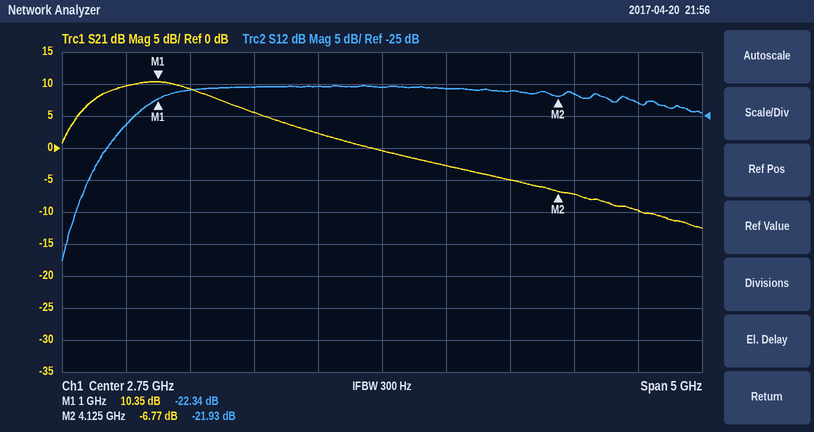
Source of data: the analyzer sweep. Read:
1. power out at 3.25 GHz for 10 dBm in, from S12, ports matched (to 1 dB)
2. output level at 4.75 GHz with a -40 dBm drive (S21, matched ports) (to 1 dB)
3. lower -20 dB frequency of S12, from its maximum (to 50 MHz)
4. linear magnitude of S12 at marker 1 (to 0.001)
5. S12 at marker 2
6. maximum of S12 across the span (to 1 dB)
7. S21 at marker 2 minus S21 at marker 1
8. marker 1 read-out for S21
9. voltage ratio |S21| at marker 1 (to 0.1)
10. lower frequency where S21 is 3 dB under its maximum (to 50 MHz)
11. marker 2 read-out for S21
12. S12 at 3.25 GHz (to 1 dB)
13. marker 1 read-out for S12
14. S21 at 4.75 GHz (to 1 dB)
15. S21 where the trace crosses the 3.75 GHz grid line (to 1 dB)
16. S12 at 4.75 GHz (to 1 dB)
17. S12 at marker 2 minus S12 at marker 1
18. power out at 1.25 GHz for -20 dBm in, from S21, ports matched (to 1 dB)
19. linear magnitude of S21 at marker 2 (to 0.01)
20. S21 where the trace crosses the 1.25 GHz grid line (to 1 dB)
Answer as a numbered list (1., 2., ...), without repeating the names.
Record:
1. -11 dBm
2. -50 dBm
3. 350 MHz
4. 0.076
5. -21.93 dB
6. -20 dB
7. -17.12 dB
8. 10.35 dB
9. 3.3
10. 500 MHz
11. -6.77 dB
12. -21 dB
13. -22.34 dB
14. -10 dB
15. -5 dB
16. -23 dB
17. 0.41 dB
18. -11 dBm
19. 0.46
20. 9 dB
